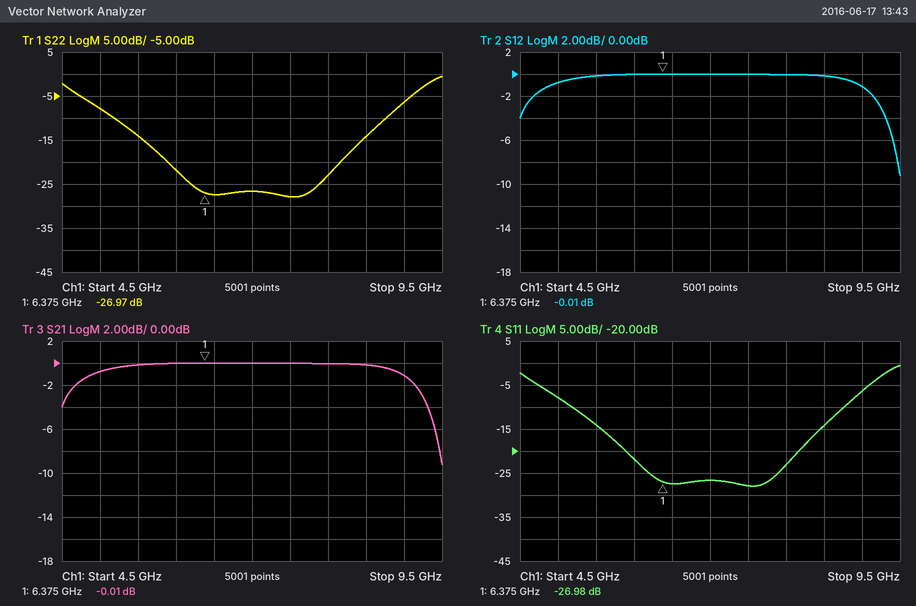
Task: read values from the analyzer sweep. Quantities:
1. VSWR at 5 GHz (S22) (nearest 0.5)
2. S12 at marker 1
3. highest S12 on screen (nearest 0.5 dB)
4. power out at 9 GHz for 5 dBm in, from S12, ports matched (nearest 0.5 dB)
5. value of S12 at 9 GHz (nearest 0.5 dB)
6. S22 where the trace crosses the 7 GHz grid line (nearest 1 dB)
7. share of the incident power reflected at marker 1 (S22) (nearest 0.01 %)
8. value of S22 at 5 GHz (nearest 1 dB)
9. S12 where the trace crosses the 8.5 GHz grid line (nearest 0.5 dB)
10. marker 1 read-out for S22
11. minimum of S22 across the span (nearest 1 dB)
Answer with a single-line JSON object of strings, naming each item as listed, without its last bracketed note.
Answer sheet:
{"VSWR at 5 GHz (S22)": "2.5", "S12 at marker 1": "-0.01 dB", "highest S12 on screen": "0.0 dB", "power out at 9 GHz for 5 dBm in, from S12, ports matched": "4.0 dBm", "value of S12 at 9 GHz": "-1.0 dB", "S22 where the trace crosses the 7 GHz grid line": "-27 dB", "share of the incident power reflected at marker 1 (S22)": "0.20 %", "value of S22 at 5 GHz": "-8 dB", "S12 where the trace crosses the 8.5 GHz grid line": "0.0 dB", "marker 1 read-out for S22": "-26.97 dB", "minimum of S22 across the span": "-28 dB"}
